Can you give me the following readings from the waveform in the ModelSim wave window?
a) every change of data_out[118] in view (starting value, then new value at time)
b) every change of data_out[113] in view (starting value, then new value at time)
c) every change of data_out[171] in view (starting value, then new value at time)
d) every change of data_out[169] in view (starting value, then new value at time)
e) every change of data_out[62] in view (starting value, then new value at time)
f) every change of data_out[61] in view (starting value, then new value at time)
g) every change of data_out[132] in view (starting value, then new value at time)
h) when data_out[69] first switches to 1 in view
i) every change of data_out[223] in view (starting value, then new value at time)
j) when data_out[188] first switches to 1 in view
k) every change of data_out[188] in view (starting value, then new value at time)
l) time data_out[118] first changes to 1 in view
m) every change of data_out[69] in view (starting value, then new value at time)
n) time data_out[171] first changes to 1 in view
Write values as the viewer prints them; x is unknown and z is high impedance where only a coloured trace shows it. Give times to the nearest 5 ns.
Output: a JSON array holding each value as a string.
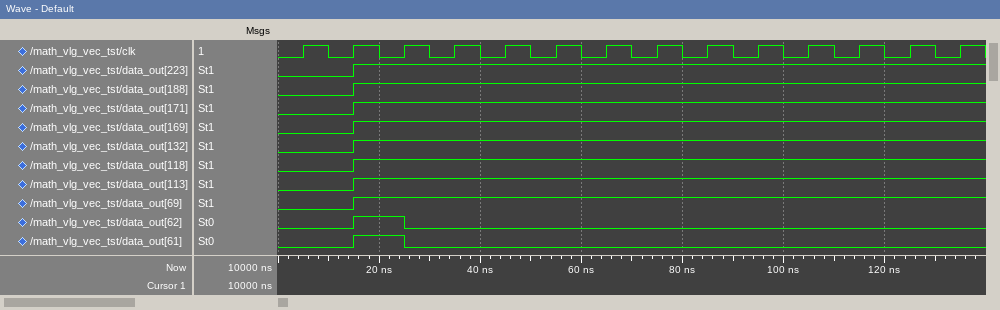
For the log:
["0, 1 at 15 ns", "0, 1 at 15 ns", "0, 1 at 15 ns", "0, 1 at 15 ns", "0, 1 at 15 ns, 0 at 25 ns", "0, 1 at 15 ns, 0 at 25 ns", "0, 1 at 15 ns", "15 ns", "0, 1 at 15 ns", "15 ns", "0, 1 at 15 ns", "15 ns", "0, 1 at 15 ns", "15 ns"]
